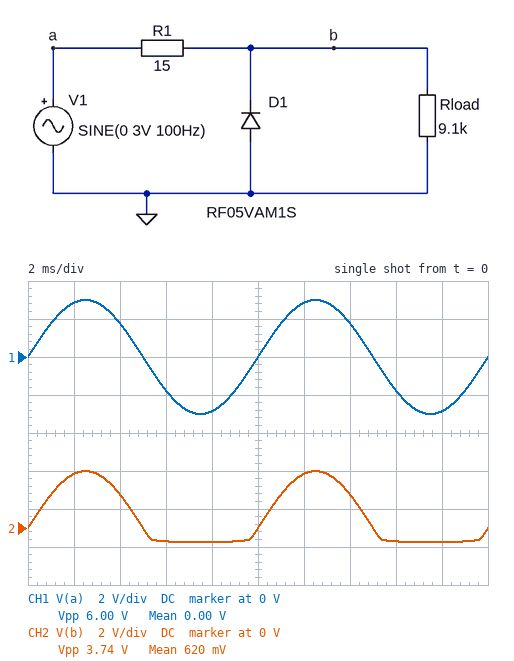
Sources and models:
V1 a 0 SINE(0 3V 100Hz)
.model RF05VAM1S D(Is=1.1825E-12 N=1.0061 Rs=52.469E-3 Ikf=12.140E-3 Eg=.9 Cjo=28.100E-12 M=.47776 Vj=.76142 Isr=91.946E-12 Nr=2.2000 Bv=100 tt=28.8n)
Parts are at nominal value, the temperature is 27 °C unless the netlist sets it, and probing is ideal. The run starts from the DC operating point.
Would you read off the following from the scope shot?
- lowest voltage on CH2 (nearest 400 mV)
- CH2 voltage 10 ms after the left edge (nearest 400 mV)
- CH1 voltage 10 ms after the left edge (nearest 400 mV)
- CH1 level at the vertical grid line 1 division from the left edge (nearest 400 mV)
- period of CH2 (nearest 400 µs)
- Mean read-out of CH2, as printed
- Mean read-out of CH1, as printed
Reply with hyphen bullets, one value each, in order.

- -800 mV
- 0 V
- 0 V
- 2.8 V
- 10.0 ms
- 620 mV
- 0.00 V
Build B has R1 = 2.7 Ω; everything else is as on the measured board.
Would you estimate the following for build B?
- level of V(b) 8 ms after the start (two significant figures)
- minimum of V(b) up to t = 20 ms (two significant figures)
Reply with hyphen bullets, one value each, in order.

- -850 mV
- -860 mV
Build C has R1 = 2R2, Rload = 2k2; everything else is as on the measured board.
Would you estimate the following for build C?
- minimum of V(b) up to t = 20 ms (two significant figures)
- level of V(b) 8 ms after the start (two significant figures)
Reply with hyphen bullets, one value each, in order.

- -880 mV
- -870 mV
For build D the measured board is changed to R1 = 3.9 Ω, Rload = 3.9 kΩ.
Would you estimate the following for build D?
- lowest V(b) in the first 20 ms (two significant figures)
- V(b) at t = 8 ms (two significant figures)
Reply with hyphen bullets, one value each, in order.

- -830 mV
- -820 mV
